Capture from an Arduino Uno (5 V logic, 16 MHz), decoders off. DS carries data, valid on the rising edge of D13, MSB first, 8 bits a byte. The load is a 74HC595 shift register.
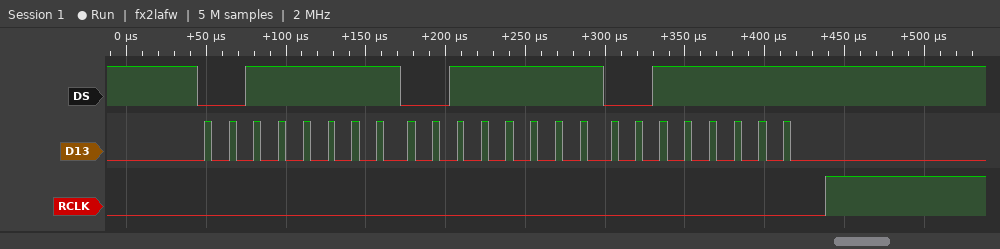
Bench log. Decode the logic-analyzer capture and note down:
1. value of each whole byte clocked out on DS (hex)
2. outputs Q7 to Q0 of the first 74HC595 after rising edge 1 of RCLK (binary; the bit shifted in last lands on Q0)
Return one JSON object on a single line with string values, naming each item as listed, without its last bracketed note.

{"value of each whole byte clocked out on DS": "0x3F 0x3F 0x3F", "outputs Q7 to Q0 of the first 74HC595 after rising edge 1 of RCLK": "00111111"}
